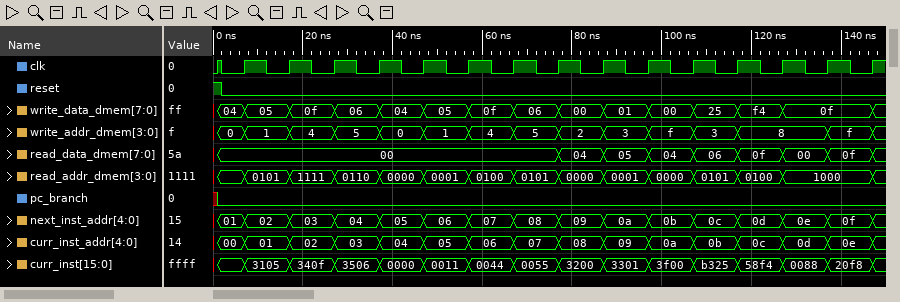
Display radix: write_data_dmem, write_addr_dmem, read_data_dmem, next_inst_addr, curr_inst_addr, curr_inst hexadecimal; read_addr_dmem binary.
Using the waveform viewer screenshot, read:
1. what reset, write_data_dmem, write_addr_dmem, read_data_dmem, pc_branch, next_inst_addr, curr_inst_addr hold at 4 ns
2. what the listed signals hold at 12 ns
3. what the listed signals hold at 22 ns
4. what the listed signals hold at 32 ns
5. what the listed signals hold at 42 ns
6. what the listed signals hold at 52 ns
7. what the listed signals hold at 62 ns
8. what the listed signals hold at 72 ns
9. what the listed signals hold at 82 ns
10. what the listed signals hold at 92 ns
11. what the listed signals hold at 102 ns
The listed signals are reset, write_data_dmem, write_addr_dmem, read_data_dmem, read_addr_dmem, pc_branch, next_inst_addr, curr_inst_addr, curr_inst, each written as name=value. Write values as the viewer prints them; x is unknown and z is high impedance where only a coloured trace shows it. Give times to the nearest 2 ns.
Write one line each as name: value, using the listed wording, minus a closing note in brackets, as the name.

what reset, write_data_dmem, write_addr_dmem, read_data_dmem, pc_branch, next_inst_addr, curr_inst_addr hold at 4 ns: reset=0, write_data_dmem=04, write_addr_dmem=0, read_data_dmem=00, pc_branch=0, next_inst_addr=01, curr_inst_addr=00
what the listed signals hold at 12 ns: reset=0, write_data_dmem=05, write_addr_dmem=1, read_data_dmem=00, read_addr_dmem=0101, pc_branch=0, next_inst_addr=02, curr_inst_addr=01, curr_inst=3105
what the listed signals hold at 22 ns: reset=0, write_data_dmem=0f, write_addr_dmem=4, read_data_dmem=00, read_addr_dmem=1111, pc_branch=0, next_inst_addr=03, curr_inst_addr=02, curr_inst=340f
what the listed signals hold at 32 ns: reset=0, write_data_dmem=06, write_addr_dmem=5, read_data_dmem=00, read_addr_dmem=0110, pc_branch=0, next_inst_addr=04, curr_inst_addr=03, curr_inst=3506
what the listed signals hold at 42 ns: reset=0, write_data_dmem=04, write_addr_dmem=0, read_data_dmem=00, read_addr_dmem=0000, pc_branch=0, next_inst_addr=05, curr_inst_addr=04, curr_inst=0000
what the listed signals hold at 52 ns: reset=0, write_data_dmem=05, write_addr_dmem=1, read_data_dmem=00, read_addr_dmem=0001, pc_branch=0, next_inst_addr=06, curr_inst_addr=05, curr_inst=0011
what the listed signals hold at 62 ns: reset=0, write_data_dmem=0f, write_addr_dmem=4, read_data_dmem=00, read_addr_dmem=0100, pc_branch=0, next_inst_addr=07, curr_inst_addr=06, curr_inst=0044
what the listed signals hold at 72 ns: reset=0, write_data_dmem=06, write_addr_dmem=5, read_data_dmem=00, read_addr_dmem=0101, pc_branch=0, next_inst_addr=08, curr_inst_addr=07, curr_inst=0055
what the listed signals hold at 82 ns: reset=0, write_data_dmem=00, write_addr_dmem=2, read_data_dmem=04, read_addr_dmem=0000, pc_branch=0, next_inst_addr=09, curr_inst_addr=08, curr_inst=3200
what the listed signals hold at 92 ns: reset=0, write_data_dmem=01, write_addr_dmem=3, read_data_dmem=05, read_addr_dmem=0001, pc_branch=0, next_inst_addr=0a, curr_inst_addr=09, curr_inst=3301
what the listed signals hold at 102 ns: reset=0, write_data_dmem=00, write_addr_dmem=f, read_data_dmem=04, read_addr_dmem=0000, pc_branch=0, next_inst_addr=0b, curr_inst_addr=0a, curr_inst=3f00
